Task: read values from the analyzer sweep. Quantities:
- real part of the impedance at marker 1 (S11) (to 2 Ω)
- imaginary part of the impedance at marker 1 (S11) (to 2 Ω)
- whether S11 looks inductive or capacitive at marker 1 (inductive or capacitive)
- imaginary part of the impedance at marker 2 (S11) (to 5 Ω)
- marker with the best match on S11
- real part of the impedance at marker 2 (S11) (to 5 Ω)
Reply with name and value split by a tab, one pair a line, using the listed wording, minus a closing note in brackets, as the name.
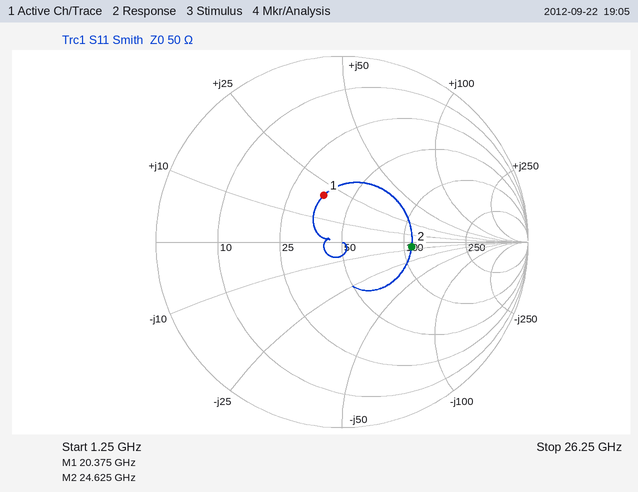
real part of the impedance at marker 1 (S11)	36 Ω
imaginary part of the impedance at marker 1 (S11)	+20 Ω
whether S11 looks inductive or capacitive at marker 1	inductive
imaginary part of the impedance at marker 2 (S11)	-5 Ω
marker with the best match on S11	marker 1
real part of the impedance at marker 2 (S11)	110 Ω
